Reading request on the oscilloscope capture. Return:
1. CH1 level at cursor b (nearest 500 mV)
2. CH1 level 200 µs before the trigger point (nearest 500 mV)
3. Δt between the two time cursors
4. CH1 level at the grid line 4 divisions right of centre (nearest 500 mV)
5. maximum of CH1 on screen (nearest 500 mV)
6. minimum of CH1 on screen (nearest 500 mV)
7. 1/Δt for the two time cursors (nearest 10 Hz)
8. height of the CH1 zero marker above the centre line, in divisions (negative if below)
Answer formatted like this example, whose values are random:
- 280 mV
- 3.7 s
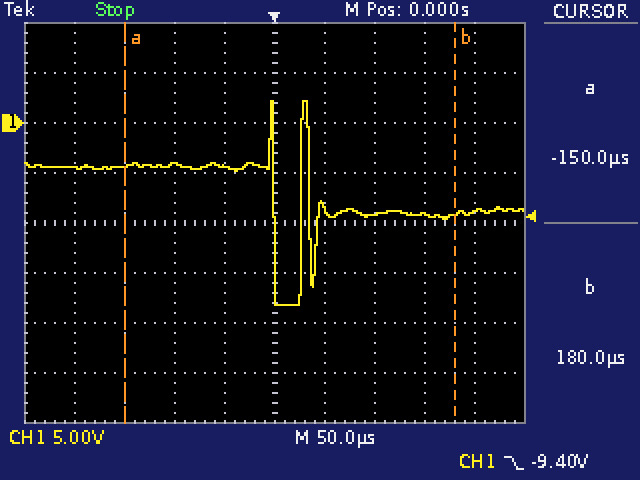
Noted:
- -9.0 V
- -4.5 V
- 330 µs
- -9.0 V
- 2.0 V
- -18.0 V
- 3.03 kHz
- +2.0 div
